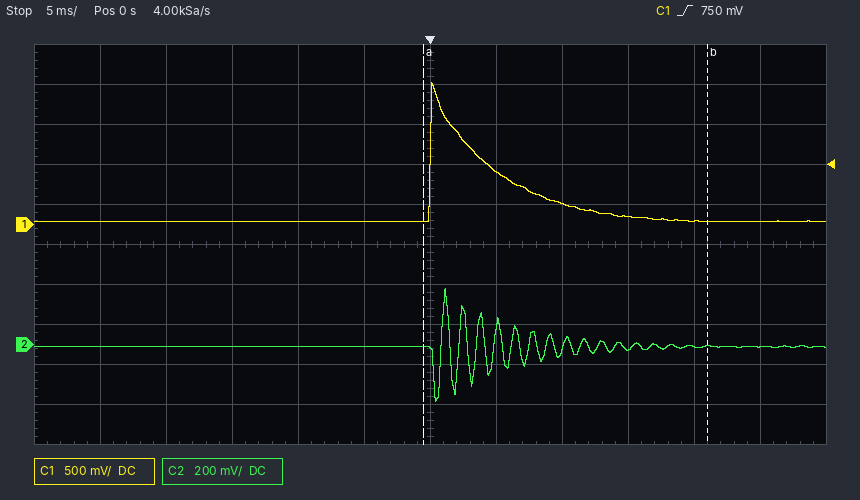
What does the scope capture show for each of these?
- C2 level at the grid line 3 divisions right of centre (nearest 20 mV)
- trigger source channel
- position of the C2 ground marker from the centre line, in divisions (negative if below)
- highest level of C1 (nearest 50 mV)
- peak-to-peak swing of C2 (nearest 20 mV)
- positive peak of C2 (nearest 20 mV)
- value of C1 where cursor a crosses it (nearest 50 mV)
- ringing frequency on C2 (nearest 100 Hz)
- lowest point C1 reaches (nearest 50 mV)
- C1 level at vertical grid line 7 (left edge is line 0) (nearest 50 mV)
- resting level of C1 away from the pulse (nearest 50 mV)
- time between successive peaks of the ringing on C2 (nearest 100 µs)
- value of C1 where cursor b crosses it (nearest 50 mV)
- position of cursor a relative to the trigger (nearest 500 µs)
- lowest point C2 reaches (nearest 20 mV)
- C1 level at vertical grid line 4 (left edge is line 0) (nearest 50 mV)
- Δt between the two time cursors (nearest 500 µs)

-20 mV
C1
-2.5 div
1.75 V
560 mV
280 mV
50 mV
800 Hz
50 mV
650 mV
50 mV
1.3 ms
50 mV
-500 µs
-280 mV
50 mV
21.5 ms
